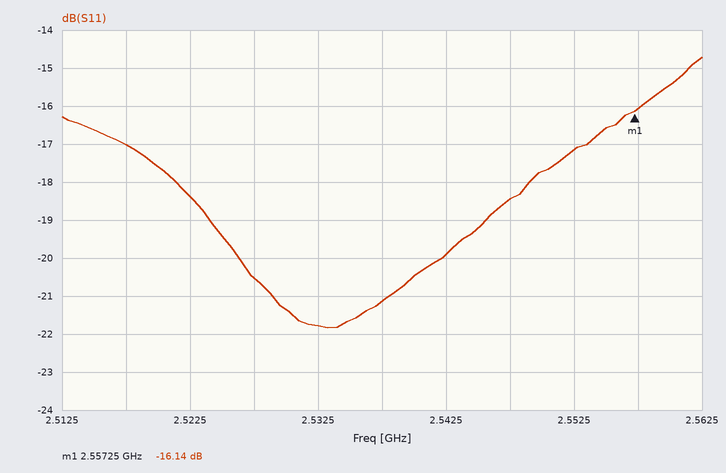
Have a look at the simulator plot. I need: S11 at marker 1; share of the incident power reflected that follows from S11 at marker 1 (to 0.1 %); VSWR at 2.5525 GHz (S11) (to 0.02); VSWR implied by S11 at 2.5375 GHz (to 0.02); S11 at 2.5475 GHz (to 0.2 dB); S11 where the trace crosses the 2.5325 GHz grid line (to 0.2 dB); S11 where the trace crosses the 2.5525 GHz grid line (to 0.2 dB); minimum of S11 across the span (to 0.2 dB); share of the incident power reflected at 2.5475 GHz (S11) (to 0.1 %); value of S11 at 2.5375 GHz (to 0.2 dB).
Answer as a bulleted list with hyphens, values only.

- -16.14 dB
- 2.4 %
- 1.32
- 1.20
- -18.4 dB
- -21.8 dB
- -17.2 dB
- -21.8 dB
- 1.4 %
- -21.2 dB
